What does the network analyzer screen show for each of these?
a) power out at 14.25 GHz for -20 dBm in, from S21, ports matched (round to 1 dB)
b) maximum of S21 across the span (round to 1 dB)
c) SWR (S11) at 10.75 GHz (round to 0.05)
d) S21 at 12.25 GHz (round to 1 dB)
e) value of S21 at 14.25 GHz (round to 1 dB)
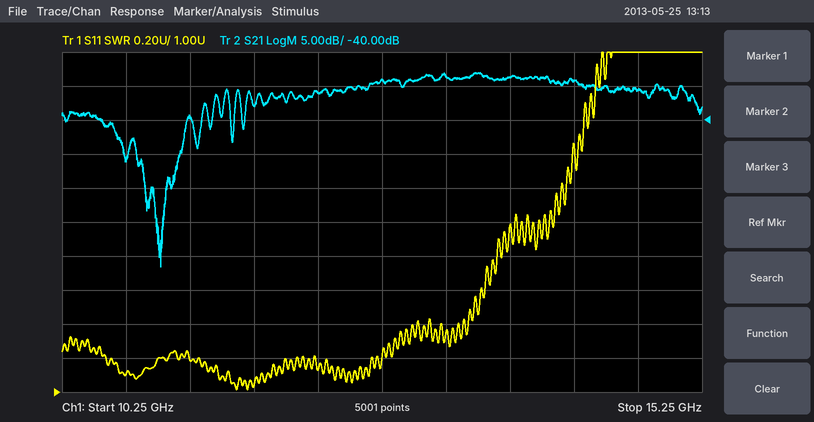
-54 dBm
-33 dB
1.10
-36 dB
-34 dB
